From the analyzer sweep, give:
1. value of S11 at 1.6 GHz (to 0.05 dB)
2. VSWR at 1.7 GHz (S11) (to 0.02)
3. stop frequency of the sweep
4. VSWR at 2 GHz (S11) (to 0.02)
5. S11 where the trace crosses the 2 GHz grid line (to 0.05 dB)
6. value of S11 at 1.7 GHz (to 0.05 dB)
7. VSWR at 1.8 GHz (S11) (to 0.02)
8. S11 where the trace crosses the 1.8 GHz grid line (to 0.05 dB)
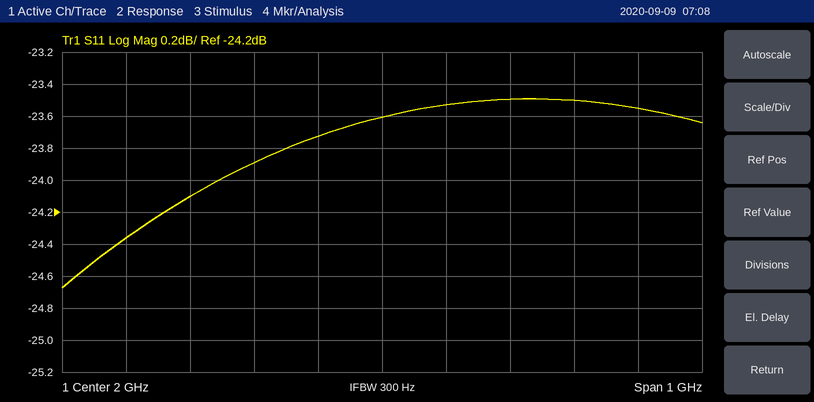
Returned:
-24.35 dB
1.14
2.5 GHz
1.14
-23.60 dB
-24.10 dB
1.14
-23.90 dB
